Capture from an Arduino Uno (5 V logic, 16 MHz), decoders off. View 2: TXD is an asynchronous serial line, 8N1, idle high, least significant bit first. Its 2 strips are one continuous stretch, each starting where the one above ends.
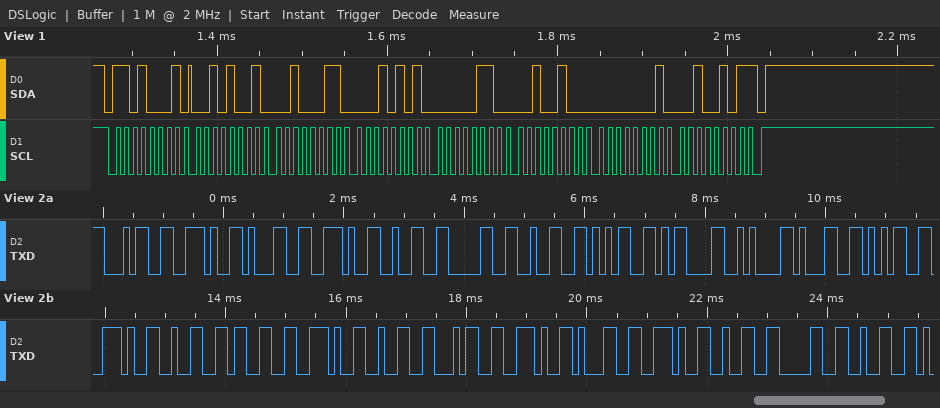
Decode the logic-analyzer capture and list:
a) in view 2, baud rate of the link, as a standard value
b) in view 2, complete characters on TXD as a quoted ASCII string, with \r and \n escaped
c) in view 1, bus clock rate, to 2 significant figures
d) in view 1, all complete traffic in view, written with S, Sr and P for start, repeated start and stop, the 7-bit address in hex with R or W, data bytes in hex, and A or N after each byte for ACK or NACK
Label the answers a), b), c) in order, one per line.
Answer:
a) 9600 baud
b) "4.1.2025\r\n15.23.24.1.202"
c) 100 kHz
d) S 68R A 29 A 23 A 15 A 06 A 24 A 01 A 25 N P
